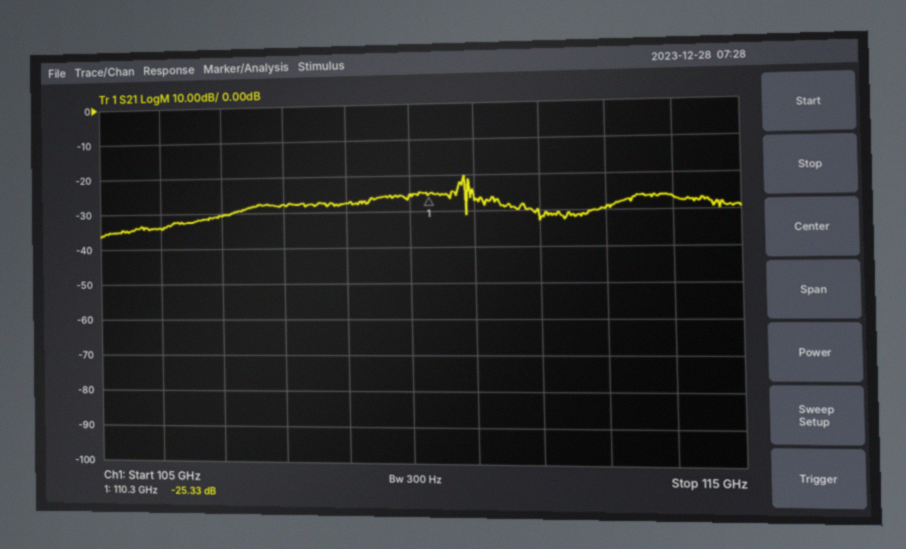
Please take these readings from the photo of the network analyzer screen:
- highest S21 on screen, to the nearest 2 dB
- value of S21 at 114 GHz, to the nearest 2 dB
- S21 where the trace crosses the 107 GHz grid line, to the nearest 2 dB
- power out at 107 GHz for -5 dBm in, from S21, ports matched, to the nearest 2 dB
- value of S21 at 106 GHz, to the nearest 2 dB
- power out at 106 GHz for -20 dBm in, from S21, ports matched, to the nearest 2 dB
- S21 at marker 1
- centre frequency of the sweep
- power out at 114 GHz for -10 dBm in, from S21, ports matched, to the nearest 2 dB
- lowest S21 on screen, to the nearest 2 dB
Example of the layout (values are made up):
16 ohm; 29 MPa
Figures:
-20 dB; -26 dB; -30 dB; -36 dBm; -34 dB; -54 dBm; -25.33 dB; 110 GHz; -36 dBm; -36 dB
